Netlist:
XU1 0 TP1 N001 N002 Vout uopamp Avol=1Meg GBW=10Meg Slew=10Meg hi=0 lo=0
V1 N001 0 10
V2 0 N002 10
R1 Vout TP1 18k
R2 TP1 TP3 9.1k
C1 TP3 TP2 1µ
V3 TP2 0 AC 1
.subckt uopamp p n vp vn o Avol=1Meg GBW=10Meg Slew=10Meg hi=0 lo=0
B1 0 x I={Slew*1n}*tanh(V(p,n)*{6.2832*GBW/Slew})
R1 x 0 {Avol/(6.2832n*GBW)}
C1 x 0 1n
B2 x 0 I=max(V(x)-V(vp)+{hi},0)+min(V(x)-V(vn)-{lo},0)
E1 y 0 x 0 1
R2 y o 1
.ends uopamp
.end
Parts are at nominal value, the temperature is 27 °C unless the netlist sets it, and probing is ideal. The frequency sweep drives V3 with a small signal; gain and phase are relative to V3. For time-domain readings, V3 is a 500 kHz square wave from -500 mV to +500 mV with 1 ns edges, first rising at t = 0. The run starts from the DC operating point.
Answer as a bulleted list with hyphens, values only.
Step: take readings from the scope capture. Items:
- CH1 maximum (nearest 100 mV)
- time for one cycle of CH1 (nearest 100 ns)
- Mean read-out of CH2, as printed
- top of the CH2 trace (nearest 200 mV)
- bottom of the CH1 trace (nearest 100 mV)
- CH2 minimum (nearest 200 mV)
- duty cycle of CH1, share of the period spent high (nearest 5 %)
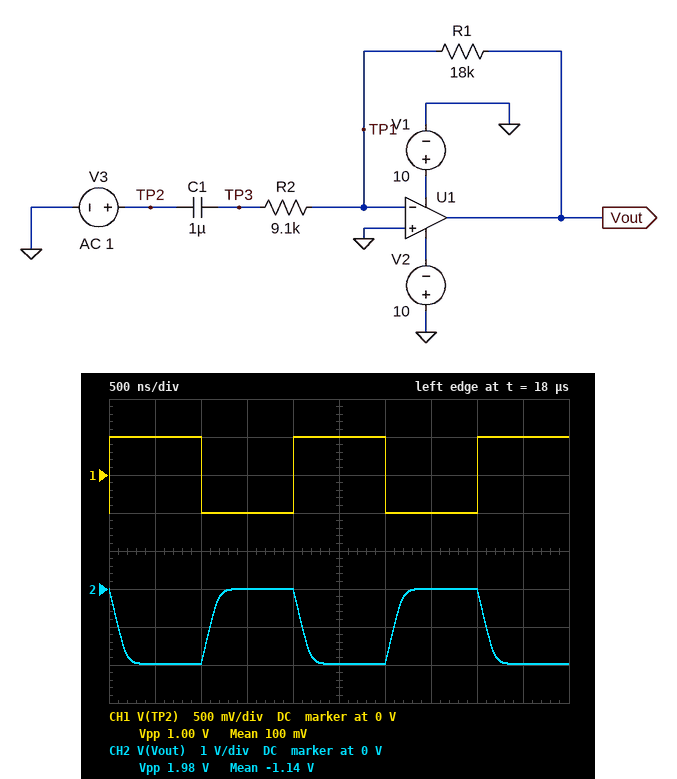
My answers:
- 500 mV
- 2.0 µs
- -1.14 V
- 0 V
- -500 mV
- -2.0 V
- 50 %
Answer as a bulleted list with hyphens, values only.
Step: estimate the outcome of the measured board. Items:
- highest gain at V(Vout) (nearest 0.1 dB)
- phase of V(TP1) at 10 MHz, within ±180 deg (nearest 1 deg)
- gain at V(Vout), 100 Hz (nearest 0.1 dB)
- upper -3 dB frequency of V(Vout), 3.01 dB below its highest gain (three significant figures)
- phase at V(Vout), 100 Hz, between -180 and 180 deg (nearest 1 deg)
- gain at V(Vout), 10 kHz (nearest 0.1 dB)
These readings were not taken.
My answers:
- 5.9 dB
- 19 deg
- 5.8 dB
- 3.36 MHz
- -170 deg
- 5.9 dB
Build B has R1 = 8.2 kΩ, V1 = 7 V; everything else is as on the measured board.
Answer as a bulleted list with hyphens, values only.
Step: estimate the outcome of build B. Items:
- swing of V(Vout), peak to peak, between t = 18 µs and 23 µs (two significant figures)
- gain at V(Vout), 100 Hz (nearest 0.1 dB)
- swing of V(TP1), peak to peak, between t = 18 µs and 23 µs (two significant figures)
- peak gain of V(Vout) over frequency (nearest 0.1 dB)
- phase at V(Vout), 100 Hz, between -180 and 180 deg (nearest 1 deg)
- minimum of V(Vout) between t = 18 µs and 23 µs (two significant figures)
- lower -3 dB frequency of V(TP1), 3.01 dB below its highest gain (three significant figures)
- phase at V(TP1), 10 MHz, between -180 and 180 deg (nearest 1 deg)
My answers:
- 900 mV
- -1.0 dB
- 940 mV
- -0.9 dB
- -170 deg
- -900 mV
- 5.26 MHz
- 28 deg
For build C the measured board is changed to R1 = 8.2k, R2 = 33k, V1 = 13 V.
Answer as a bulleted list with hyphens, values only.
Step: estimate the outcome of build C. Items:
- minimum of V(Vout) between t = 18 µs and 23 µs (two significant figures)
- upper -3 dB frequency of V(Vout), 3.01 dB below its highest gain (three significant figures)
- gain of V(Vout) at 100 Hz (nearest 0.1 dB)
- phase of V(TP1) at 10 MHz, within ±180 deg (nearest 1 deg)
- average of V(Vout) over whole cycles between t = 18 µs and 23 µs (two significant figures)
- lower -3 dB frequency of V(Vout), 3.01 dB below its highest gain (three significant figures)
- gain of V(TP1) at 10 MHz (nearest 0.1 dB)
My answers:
- -250 mV
- 8.01 MHz
- -12.1 dB
- 39 deg
- -120 mV
- 4.82 Hz
- -16.2 dB
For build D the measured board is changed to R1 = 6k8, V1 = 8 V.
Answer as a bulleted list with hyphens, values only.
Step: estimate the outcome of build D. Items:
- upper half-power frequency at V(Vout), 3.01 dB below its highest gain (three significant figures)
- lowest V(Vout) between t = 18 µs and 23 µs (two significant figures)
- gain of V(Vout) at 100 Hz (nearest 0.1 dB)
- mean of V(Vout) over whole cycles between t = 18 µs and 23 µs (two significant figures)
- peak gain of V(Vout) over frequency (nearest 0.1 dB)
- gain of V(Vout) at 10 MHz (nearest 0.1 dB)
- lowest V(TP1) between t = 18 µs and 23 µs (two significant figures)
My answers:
- 5.72 MHz
- -750 mV
- -2.7 dB
- -370 mV
- -2.5 dB
- -8.6 dB
- -420 mV
